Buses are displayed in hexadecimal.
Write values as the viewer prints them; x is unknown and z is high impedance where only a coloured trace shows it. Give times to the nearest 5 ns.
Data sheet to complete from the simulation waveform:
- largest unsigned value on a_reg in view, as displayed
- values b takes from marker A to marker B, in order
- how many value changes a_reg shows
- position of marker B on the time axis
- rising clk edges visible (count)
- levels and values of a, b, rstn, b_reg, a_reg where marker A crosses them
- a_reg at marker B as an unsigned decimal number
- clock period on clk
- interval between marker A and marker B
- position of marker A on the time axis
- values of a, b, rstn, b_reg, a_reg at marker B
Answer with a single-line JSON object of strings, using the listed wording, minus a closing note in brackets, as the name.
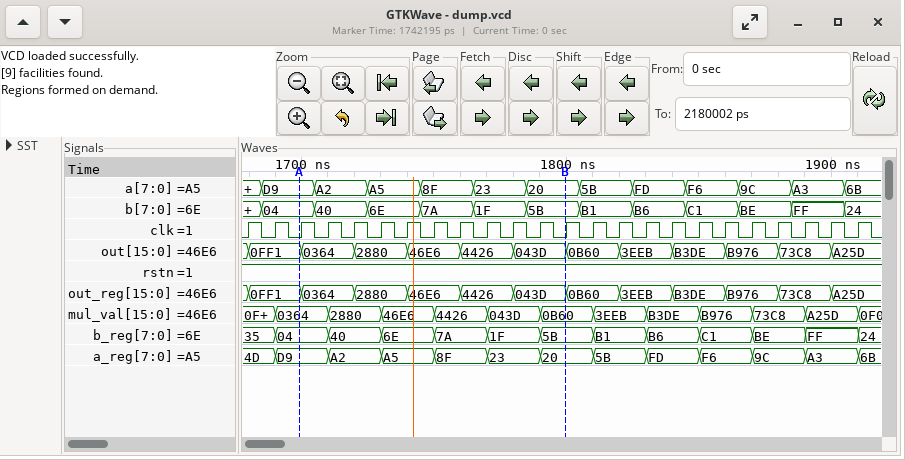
{"largest unsigned value on a_reg in view, as displayed": "FD", "values b takes from marker A to marker B, in order": "04, 40, 6E, 7A, 1F, 5B", "how many value changes a_reg shows": "12", "position of marker B on the time axis": "1800 ns", "rising clk edges visible": "24", "levels and values of a, b, rstn, b_reg, a_reg where marker A crosses them": "a=D9, b=04, rstn=1, b_reg=04, a_reg=D9", "a_reg at marker B as an unsigned decimal number": "32", "clock period on clk": "10 ns", "interval between marker A and marker B": "100 ns", "position of marker A on the time axis": "1700 ns", "values of a, b, rstn, b_reg, a_reg at marker B": "a=20, b=5B, rstn=1, b_reg=5B, a_reg=20"}
